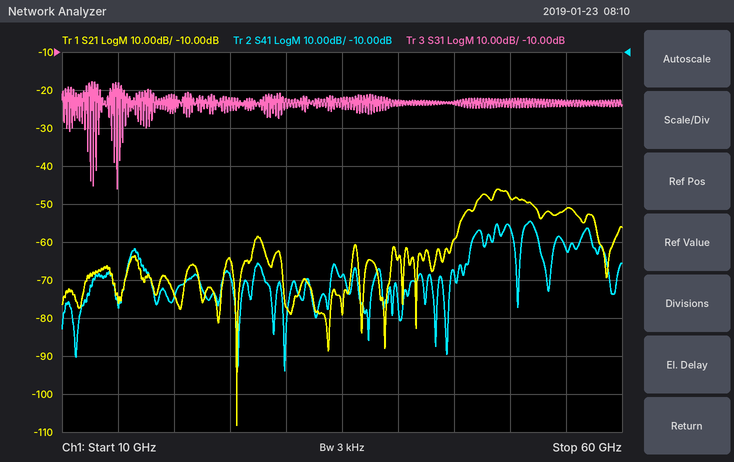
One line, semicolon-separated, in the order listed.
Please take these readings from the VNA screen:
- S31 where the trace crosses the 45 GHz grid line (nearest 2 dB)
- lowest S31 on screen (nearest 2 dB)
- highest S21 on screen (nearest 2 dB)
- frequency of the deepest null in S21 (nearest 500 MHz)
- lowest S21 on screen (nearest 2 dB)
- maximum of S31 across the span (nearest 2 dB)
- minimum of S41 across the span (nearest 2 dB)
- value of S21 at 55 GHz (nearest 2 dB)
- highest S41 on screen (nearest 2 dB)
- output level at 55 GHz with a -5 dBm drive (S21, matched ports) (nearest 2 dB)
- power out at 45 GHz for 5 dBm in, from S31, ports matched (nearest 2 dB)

-24 dB; -46 dB; -46 dB; 25.5 GHz; -108 dB; -18 dB; -94 dB; -52 dB; -54 dB; -56 dBm; -18 dBm
